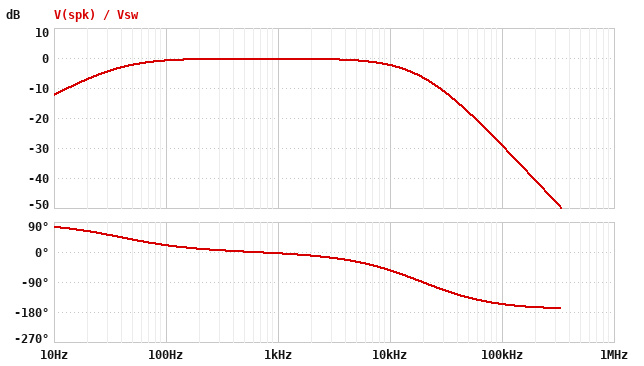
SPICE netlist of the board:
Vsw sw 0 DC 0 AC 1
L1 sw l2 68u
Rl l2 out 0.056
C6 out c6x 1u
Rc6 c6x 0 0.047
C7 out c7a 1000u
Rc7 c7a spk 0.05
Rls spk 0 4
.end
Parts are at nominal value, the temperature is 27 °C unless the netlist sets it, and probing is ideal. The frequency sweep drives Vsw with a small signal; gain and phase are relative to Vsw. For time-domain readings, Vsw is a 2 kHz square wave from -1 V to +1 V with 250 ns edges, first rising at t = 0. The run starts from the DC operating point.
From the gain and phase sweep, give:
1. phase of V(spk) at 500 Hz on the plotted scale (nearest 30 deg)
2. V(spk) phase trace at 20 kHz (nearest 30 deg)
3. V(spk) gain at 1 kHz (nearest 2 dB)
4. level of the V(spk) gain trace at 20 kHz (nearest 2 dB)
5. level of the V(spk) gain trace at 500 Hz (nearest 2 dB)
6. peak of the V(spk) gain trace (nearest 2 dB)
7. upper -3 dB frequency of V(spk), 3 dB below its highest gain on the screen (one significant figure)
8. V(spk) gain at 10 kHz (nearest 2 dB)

0 deg
-90 deg
0 dB
-6 dB
0 dB
0 dB
10 kHz
-2 dB
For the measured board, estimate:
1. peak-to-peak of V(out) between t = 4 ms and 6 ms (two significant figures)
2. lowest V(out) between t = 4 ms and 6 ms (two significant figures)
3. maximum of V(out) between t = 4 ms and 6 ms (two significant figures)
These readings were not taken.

2.0 V
-990 mV
990 mV
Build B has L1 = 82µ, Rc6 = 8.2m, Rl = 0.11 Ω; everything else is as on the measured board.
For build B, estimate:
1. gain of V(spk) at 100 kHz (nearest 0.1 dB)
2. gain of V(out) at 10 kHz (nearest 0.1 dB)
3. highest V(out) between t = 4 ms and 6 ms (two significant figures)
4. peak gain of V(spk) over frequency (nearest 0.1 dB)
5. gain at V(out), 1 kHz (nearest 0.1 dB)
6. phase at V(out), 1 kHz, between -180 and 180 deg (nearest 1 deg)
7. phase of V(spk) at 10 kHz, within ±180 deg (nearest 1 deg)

-30.7 dB
-3.3 dB
970 mV
-0.3 dB
-0.2 dB
-7 deg
-61 deg
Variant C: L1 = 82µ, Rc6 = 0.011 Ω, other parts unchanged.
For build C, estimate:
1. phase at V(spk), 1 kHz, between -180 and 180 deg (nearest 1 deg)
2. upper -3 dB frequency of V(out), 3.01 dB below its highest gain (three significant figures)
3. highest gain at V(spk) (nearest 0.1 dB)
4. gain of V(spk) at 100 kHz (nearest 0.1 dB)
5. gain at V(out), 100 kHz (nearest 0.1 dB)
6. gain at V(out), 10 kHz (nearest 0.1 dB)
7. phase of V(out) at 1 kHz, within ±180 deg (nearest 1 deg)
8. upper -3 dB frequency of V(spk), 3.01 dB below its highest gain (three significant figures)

-5 deg
9.58 kHz
-0.2 dB
-30.7 dB
-30.6 dB
-3.2 dB
-7 deg
9.80 kHz
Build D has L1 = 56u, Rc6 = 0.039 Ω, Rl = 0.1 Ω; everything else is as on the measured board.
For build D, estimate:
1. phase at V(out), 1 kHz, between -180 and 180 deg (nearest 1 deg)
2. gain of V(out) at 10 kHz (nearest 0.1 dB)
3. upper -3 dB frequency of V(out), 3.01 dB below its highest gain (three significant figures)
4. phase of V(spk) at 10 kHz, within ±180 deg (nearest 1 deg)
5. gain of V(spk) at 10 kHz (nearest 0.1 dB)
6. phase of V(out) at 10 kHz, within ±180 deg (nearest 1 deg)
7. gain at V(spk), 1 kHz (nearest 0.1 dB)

-5 deg
-1.5 dB
15.0 kHz
-47 deg
-1.6 dB
-48 deg
-0.3 dB
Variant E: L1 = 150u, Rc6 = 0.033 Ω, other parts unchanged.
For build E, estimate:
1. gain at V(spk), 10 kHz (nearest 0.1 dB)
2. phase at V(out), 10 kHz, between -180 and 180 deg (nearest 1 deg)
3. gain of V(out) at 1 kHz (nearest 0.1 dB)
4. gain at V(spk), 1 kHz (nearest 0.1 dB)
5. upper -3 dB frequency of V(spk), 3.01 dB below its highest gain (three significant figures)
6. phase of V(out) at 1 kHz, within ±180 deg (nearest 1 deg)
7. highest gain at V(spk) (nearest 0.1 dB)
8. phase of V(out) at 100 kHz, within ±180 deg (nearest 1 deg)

-7.6 dB
-80 deg
-0.2 dB
-0.3 dB
4.91 kHz
-13 deg
-0.2 dB
-157 deg
